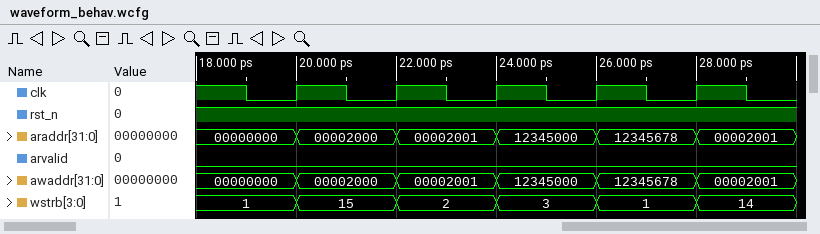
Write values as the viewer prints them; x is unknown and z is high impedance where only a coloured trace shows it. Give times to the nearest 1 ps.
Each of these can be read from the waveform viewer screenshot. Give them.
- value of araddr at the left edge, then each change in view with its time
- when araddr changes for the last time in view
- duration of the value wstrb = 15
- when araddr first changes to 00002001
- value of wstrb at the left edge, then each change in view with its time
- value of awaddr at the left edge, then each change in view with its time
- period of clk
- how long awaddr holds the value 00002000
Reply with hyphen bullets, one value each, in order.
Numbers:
- 00000000, 00002000 at 20 ps, 00002001 at 22 ps, 12345000 at 24 ps, 12345678 at 26 ps, 00002001 at 28 ps
- 28 ps
- 2 ps
- 22 ps
- 1, 15 at 20 ps, 2 at 22 ps, 3 at 24 ps, 1 at 26 ps, 14 at 28 ps
- 00000000, 00002000 at 20 ps, 00002001 at 22 ps, 12345000 at 24 ps, 12345678 at 26 ps, 00002001 at 28 ps
- 2 ps
- 2 ps
